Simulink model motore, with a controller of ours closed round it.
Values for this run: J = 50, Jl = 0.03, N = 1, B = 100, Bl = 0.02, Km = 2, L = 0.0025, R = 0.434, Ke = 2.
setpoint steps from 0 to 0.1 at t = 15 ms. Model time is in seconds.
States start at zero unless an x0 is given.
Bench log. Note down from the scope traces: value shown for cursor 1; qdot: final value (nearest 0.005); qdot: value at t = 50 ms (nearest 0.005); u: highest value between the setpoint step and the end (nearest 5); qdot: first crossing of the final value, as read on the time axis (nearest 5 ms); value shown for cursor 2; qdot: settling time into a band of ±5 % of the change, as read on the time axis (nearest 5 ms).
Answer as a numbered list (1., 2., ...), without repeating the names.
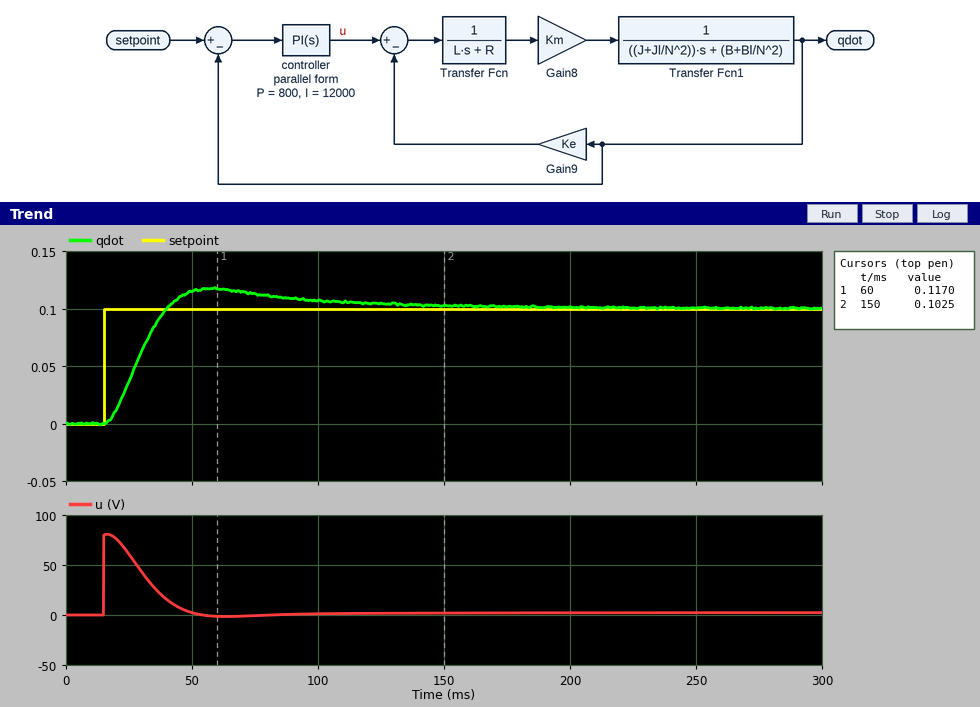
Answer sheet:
1. 0.1170
2. 0.100
3. 0.115
4. 80
5. 40 ms
6. 0.1025
7. 115 ms
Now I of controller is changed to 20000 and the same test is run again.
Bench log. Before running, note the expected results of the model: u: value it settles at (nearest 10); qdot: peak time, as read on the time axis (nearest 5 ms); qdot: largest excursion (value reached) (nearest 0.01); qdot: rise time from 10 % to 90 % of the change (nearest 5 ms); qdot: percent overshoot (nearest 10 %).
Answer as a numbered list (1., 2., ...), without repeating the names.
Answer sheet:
1. 0
2. 55 ms
3. 0.13
4. 15 ms
5. 30 %
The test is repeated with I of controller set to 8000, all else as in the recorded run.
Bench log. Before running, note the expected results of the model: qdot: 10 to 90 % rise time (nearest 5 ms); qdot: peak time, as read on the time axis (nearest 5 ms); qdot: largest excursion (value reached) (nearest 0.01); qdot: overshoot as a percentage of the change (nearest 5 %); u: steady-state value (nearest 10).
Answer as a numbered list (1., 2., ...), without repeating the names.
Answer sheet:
1. 20 ms
2. 60 ms
3. 0.11
4. 10 %
5. 0
